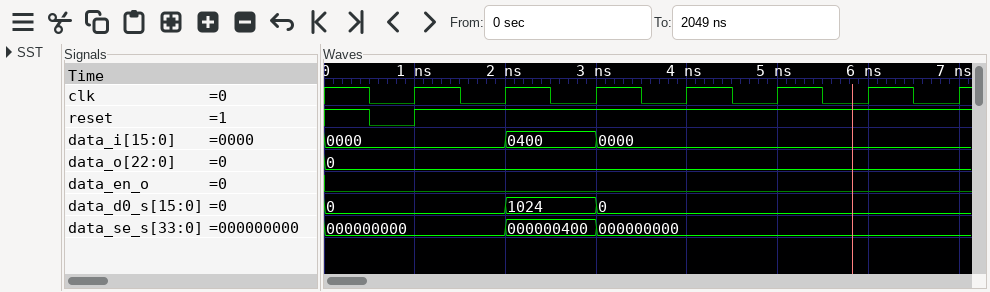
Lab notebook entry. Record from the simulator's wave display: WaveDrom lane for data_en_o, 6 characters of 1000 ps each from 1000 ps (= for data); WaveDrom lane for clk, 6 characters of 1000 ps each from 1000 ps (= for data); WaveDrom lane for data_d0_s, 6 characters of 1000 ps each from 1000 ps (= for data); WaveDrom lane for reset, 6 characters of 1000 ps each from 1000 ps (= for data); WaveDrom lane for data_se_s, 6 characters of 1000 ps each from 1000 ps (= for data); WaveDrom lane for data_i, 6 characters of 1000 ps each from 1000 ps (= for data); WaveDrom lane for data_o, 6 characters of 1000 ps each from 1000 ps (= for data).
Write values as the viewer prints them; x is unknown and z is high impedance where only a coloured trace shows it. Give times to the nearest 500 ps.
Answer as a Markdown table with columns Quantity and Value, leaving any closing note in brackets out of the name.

| Quantity | Value |
|---|---|
| WaveDrom lane for data_en_o, 6 characters of 1000 ps each from 1000 ps | {name: 'data_en_o', wave: '0.....'} |
| WaveDrom lane for clk, 6 characters of 1000 ps each from 1000 ps | {name: 'clk', wave: 'p.....'} |
| WaveDrom lane for data_d0_s, 6 characters of 1000 ps each from 1000 ps | {name: 'data_d0_s', wave: '===...', data: '0 1024 0'} |
| WaveDrom lane for reset, 6 characters of 1000 ps each from 1000 ps | {name: 'reset', wave: '1.....'} |
| WaveDrom lane for data_se_s, 6 characters of 1000 ps each from 1000 ps | {name: 'data_se_s', wave: '===...', data: '000000000 000000400 000000000'} |
| WaveDrom lane for data_i, 6 characters of 1000 ps each from 1000 ps | {name: 'data_i', wave: '===...', data: '0000 0400 0000'} |
| WaveDrom lane for data_o, 6 characters of 1000 ps each from 1000 ps | {name: 'data_o', wave: '=.....', data: '0'} |
